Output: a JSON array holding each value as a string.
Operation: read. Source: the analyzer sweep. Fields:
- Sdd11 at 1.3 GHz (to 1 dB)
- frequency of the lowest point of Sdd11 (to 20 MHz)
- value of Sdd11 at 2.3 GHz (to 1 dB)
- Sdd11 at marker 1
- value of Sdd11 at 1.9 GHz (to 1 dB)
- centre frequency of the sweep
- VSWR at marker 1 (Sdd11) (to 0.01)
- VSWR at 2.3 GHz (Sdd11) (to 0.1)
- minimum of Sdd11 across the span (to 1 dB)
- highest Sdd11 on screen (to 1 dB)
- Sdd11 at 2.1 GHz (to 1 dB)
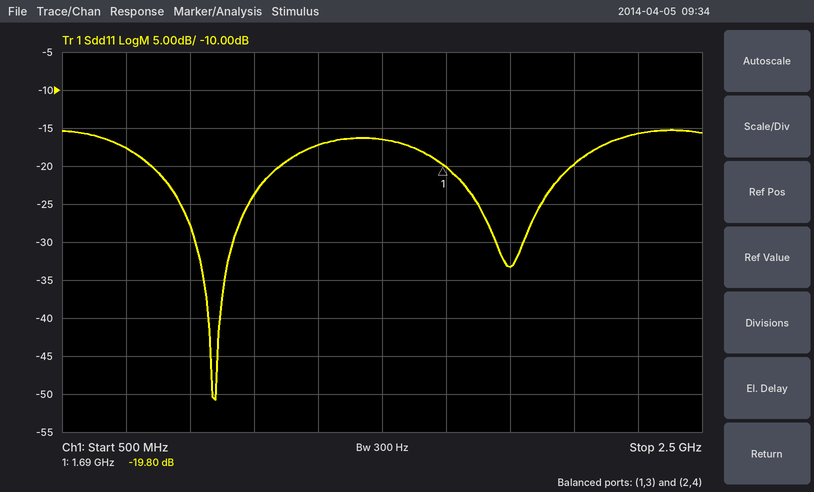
["-17 dB", "980 MHz", "-16 dB", "-19.80 dB", "-33 dB", "1.5 GHz", "1.23", "1.4", "-51 dB", "-15 dB", "-20 dB"]
